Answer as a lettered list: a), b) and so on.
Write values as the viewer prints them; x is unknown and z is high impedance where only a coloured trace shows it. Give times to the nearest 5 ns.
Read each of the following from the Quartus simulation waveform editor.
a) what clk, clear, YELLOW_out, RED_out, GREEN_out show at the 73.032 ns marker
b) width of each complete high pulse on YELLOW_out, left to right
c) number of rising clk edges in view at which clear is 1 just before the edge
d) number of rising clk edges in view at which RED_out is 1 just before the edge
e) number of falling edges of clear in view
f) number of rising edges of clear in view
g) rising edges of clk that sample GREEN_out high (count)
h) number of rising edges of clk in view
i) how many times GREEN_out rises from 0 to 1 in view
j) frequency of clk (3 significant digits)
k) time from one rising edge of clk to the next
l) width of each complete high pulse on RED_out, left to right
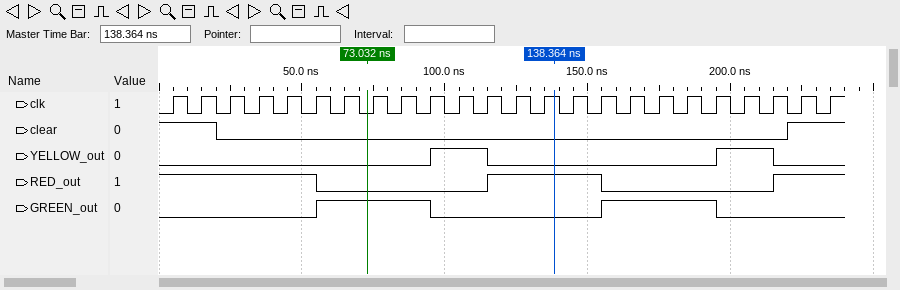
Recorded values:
a) clk=0, clear=0, YELLOW_out=0, RED_out=0, GREEN_out=1
b) 20 ns, 20 ns
c) 4
d) 12
e) 1
f) 1
g) 8
h) 24
i) 2
j) 100 MHz
k) 10 ns
l) 40 ns
